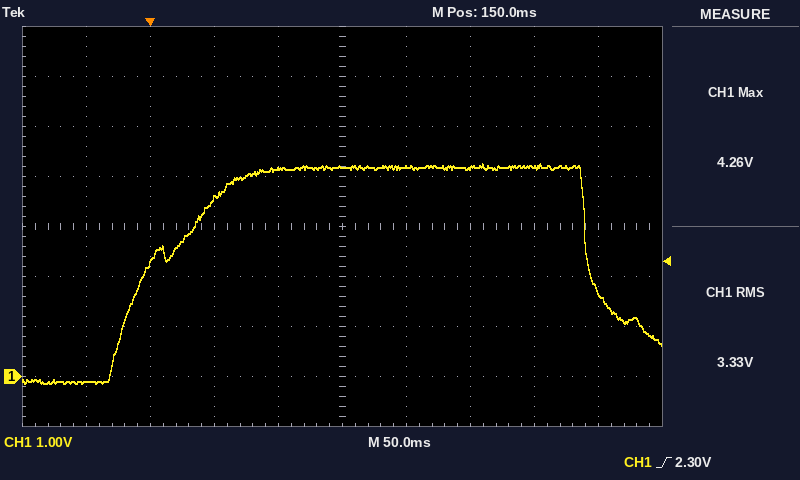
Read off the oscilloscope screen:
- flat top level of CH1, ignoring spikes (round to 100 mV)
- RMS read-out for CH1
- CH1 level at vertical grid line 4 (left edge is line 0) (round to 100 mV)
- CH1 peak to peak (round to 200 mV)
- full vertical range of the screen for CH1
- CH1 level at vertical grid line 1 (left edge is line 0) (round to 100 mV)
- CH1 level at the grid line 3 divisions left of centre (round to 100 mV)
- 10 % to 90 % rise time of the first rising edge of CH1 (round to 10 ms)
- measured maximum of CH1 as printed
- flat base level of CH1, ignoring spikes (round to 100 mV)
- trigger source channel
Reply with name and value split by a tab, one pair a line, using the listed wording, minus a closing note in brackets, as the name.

flat top level of CH1, ignoring spikes	4.2 V
RMS read-out for CH1	3.33 V
CH1 level at vertical grid line 4 (left edge is line 0)	4.2 V
CH1 peak to peak	4.4 V
full vertical range of the screen for CH1	8 V
CH1 level at vertical grid line 1 (left edge is line 0)	-100 mV
CH1 level at the grid line 3 divisions left of centre	2.3 V
10 % to 90 % rise time of the first rising edge of CH1	90 ms
measured maximum of CH1 as printed	4.26 V
flat base level of CH1, ignoring spikes	-100 mV
trigger source channel	CH1
